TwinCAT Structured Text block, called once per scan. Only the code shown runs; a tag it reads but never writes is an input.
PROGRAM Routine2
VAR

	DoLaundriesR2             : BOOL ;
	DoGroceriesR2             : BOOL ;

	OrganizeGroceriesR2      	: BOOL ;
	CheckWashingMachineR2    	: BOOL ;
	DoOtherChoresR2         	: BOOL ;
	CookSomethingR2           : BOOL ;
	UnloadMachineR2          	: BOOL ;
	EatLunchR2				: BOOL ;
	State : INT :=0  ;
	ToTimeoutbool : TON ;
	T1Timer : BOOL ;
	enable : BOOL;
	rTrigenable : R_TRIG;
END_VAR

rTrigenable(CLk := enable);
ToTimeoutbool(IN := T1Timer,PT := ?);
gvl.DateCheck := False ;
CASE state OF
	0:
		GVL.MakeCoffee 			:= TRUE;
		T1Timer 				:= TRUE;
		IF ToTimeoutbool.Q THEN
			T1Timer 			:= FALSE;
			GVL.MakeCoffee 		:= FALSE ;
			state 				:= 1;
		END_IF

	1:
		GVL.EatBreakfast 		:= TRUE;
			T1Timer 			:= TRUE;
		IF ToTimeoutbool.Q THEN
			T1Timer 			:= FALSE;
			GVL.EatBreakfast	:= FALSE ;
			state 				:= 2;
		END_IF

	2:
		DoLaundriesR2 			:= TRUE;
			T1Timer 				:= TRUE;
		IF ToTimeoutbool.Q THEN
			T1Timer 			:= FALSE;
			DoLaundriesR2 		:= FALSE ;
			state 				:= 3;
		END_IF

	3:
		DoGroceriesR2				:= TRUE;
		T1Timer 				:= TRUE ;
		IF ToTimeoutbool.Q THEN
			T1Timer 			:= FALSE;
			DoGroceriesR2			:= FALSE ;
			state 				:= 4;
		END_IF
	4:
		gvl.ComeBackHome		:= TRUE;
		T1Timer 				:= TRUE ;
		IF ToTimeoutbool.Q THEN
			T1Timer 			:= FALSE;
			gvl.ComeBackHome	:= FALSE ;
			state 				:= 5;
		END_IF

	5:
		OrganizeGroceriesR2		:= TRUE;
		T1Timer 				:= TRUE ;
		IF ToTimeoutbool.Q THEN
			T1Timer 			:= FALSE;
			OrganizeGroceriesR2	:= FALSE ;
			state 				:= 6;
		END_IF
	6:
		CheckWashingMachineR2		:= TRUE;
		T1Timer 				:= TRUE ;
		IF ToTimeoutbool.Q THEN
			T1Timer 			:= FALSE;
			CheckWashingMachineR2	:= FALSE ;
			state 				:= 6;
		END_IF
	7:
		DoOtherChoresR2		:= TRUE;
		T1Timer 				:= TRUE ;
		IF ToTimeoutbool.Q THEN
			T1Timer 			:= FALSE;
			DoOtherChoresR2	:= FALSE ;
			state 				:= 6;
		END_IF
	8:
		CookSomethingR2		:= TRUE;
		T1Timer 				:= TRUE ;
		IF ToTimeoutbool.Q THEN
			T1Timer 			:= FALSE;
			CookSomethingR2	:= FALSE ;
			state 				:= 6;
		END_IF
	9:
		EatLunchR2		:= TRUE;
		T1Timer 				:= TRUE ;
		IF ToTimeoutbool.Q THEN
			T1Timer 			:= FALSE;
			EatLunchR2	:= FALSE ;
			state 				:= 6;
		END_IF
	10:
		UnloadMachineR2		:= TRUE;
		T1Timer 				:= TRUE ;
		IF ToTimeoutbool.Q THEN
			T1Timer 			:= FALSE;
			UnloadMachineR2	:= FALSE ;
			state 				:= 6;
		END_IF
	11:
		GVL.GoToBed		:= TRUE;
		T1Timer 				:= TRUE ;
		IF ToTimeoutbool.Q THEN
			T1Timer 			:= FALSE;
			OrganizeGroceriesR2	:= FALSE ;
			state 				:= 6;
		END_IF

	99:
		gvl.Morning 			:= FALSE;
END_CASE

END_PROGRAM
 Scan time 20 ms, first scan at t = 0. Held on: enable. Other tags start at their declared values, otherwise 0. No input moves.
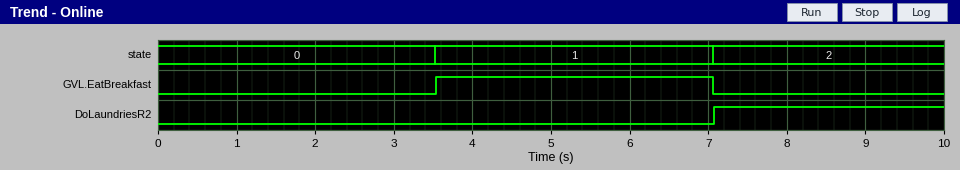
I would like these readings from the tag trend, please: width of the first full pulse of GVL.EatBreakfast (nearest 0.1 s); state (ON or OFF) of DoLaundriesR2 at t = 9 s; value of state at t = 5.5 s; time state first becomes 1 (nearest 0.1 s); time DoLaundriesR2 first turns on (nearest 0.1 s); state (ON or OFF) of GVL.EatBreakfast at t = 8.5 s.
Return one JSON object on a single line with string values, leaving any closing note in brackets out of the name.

{"width of the first full pulse of GVL.EatBreakfast": "3.5 s", "state (ON or OFF) of DoLaundriesR2 at t = 9 s": "ON", "value of state at t = 5.5 s": "1", "time state first becomes 1": "3.5 s", "time DoLaundriesR2 first turns on": "7.1 s", "state (ON or OFF) of GVL.EatBreakfast at t = 8.5 s": "OFF"}
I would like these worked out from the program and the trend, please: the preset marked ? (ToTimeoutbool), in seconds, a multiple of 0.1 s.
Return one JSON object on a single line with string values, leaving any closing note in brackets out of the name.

{"the preset marked ? (ToTimeoutbool), in seconds, a multiple of 0.1 s": "3.5 s"}
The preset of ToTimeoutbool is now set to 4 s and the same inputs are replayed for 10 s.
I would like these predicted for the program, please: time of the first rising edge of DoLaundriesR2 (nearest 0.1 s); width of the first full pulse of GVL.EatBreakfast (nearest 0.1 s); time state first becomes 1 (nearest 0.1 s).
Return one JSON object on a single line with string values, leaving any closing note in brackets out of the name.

{"time of the first rising edge of DoLaundriesR2": "8.1 s", "width of the first full pulse of GVL.EatBreakfast": "4.0 s", "time state first becomes 1": "4.0 s"}
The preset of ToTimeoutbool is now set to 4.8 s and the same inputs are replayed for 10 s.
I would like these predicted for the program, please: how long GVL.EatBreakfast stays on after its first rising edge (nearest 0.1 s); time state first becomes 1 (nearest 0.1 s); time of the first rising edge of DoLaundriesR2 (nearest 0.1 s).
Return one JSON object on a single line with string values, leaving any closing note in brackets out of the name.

{"how long GVL.EatBreakfast stays on after its first rising edge": "4.8 s", "time state first becomes 1": "4.8 s", "time of the first rising edge of DoLaundriesR2": "9.7 s"}
